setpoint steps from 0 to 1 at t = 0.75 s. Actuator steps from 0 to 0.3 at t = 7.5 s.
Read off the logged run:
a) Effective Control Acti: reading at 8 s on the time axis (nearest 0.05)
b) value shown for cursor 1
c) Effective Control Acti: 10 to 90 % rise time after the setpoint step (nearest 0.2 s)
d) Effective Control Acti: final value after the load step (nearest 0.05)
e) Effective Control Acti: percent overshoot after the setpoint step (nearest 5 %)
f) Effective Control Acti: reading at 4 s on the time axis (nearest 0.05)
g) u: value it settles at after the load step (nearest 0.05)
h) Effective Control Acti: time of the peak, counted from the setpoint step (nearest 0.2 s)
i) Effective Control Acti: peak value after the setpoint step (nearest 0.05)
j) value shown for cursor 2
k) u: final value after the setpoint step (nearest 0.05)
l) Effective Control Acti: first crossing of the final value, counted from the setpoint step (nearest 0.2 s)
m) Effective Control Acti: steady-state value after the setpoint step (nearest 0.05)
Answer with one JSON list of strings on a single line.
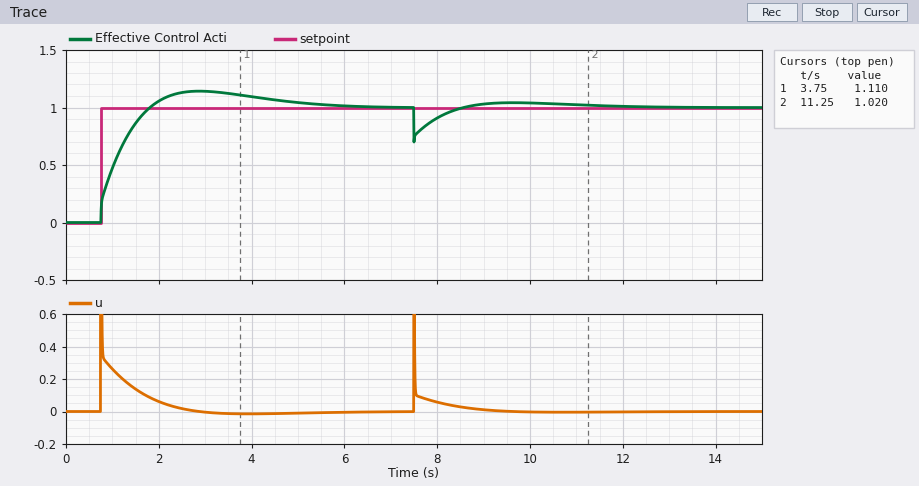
["0.90", "1.110", "0.8 s", "1.00", "15 %", "1.10", "0.00", "2.2 s", "1.15", "1.020", "0.00", "1.0 s", "1.00"]
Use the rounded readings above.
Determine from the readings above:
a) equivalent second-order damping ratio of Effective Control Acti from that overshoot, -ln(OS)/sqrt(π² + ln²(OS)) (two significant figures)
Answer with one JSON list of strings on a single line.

["0.52"]
